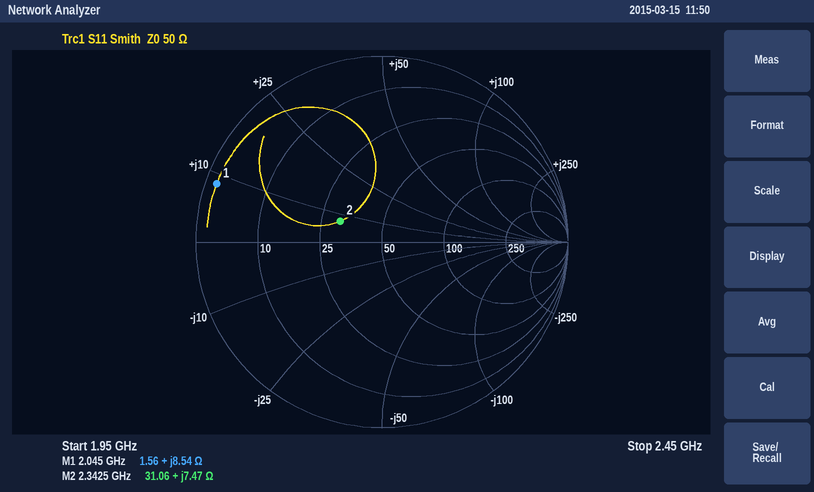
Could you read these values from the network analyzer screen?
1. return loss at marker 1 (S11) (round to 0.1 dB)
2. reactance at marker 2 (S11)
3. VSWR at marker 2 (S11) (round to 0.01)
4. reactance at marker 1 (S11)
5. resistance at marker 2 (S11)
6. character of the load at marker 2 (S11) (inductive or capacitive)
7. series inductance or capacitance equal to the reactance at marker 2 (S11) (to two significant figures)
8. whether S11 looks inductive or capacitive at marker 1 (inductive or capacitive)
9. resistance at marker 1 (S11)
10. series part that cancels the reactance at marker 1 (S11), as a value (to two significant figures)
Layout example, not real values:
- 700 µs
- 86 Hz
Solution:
- 0.5 dB
- +7.47 Ω
- 1.67
- +8.54 Ω
- 31.06 Ω
- inductive
- 510 pH
- inductive
- 1.56 Ω
- 9.1 pF
